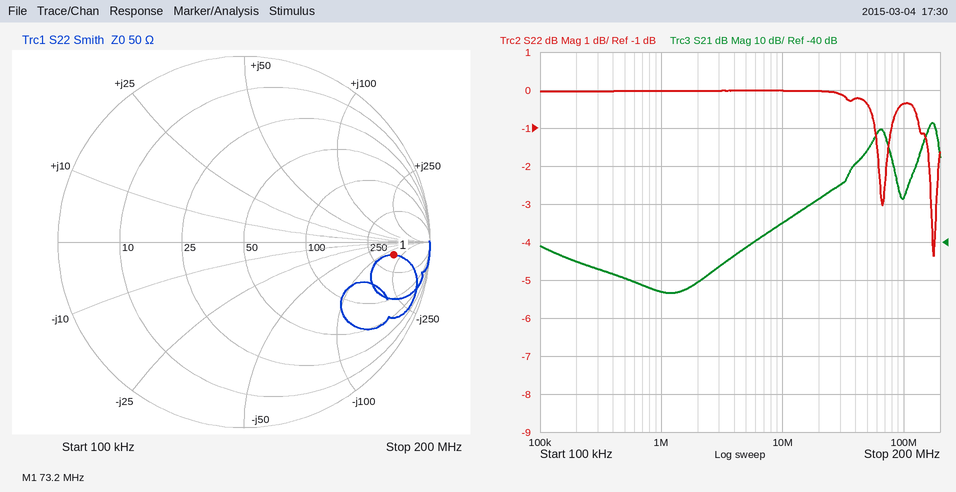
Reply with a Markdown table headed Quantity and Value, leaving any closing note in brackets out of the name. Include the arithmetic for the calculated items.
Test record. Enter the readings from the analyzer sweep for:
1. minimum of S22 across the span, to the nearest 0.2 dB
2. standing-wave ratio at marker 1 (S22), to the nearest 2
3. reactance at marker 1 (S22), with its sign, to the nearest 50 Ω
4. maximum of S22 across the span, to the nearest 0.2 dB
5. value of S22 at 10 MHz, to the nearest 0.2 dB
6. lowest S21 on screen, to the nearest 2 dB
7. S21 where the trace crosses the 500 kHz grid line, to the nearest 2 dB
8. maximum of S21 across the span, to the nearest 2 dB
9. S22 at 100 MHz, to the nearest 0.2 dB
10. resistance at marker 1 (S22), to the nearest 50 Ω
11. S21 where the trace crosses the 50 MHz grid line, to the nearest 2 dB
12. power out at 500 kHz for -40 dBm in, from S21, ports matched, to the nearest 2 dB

| Quantity | Value |
|---|---|
| minimum of S22 across the span, to the nearest 0.2 dB | -4.4 dB |
| standing-wave ratio at marker 1 (S22), to the nearest 2 | 10 |
| reactance at marker 1 (S22), with its sign, to the nearest 50 Ω | -150 Ω |
| maximum of S22 across the span, to the nearest 0.2 dB | 0.0 dB |
| value of S22 at 10 MHz, to the nearest 0.2 dB | 0.0 dB |
| lowest S21 on screen, to the nearest 2 dB | -54 dB |
| S21 where the trace crosses the 500 kHz grid line, to the nearest 2 dB | -50 dB |
| maximum of S21 across the span, to the nearest 2 dB | -8 dB |
| S22 at 100 MHz, to the nearest 0.2 dB | -0.4 dB |
| resistance at marker 1 (S22), to the nearest 50 Ω | 400 Ω |
| S21 where the trace crosses the 50 MHz grid line, to the nearest 2 dB | -16 dB |
| power out at 500 kHz for -40 dBm in, from S21, ports matched, to the nearest 2 dB | -40 dBm + (-50 dB) = -90 dBm |
